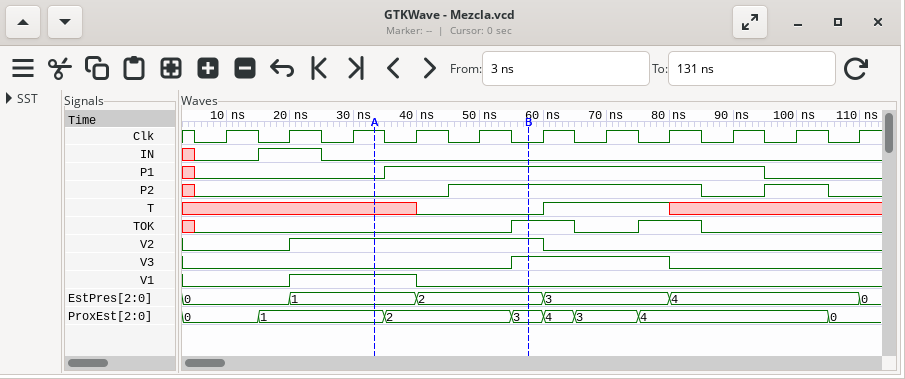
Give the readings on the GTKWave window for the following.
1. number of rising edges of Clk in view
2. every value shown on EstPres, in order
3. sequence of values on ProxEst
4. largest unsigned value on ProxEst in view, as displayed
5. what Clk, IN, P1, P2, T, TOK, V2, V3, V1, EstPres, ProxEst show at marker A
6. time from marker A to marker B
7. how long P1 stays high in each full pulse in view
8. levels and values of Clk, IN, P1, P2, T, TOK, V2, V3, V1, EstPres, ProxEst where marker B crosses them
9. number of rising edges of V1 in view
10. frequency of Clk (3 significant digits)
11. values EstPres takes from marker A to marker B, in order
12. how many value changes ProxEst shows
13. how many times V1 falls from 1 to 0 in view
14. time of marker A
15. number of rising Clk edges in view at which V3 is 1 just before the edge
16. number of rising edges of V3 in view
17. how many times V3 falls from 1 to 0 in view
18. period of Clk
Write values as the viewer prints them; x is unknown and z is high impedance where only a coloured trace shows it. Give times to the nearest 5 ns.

11
0, 1, 2, 3, 4, 0
0, 1, 2, 3, 4, 3, 4, 0
4
Clk=1, IN=0, P1=0, P2=0, T=x, TOK=0, V2=1, V3=0, V1=1, EstPres=1, ProxEst=1
25 ns
60 ns
Clk=0, IN=0, P1=1, P2=1, T=0, TOK=1, V2=1, V3=1, V1=0, EstPres=2, ProxEst=3
1
100 MHz
1, 2
7
1
35 ns
3
1
1
10 ns
